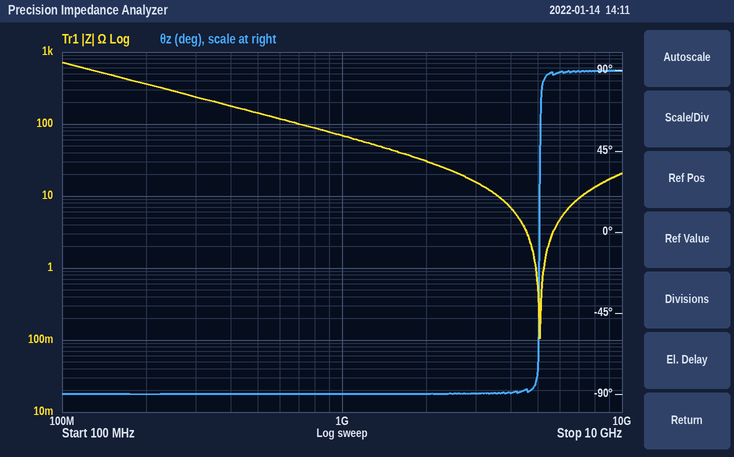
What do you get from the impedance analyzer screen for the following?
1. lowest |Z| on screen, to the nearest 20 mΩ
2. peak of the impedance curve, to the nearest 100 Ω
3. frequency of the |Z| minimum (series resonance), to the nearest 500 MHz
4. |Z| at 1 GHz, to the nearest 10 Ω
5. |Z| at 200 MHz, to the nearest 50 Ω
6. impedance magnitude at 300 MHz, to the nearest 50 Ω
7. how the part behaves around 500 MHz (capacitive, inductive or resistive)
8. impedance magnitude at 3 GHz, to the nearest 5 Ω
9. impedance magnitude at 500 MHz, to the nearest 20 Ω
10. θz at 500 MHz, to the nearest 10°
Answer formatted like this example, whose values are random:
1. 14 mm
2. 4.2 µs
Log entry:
1. 100 mΩ
2. 700 Ω
3. 5.0 GHz
4. 70 Ω
5. 350 Ω
6. 250 Ω
7. capacitive
8. 15 Ω
9. 140 Ω
10. -90°
